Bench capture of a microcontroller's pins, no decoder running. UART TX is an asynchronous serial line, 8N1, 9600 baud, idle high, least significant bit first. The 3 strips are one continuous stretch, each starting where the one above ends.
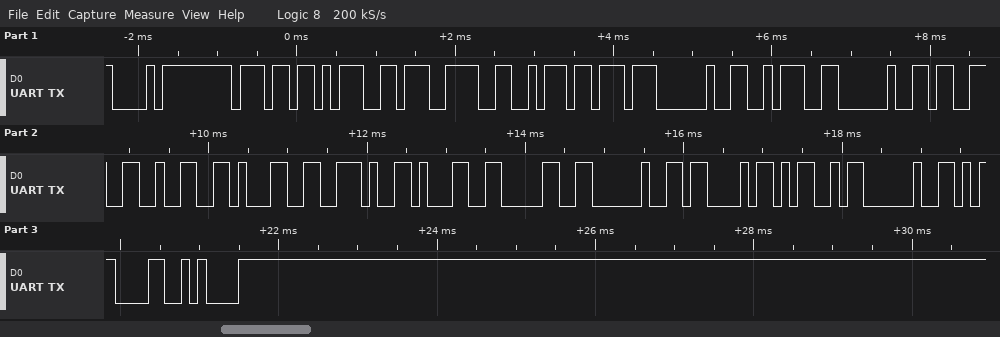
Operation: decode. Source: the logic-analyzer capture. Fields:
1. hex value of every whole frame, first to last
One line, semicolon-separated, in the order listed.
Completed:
0xE8 0xB7 0x9D 0xE7 0xA6 0xBB 0x20 0x3A 0x20 0x33 0x32 0x31 0x2E 0x31 0x30 0x20 0x43 0x4D 0x20 0x0D 0x0A
